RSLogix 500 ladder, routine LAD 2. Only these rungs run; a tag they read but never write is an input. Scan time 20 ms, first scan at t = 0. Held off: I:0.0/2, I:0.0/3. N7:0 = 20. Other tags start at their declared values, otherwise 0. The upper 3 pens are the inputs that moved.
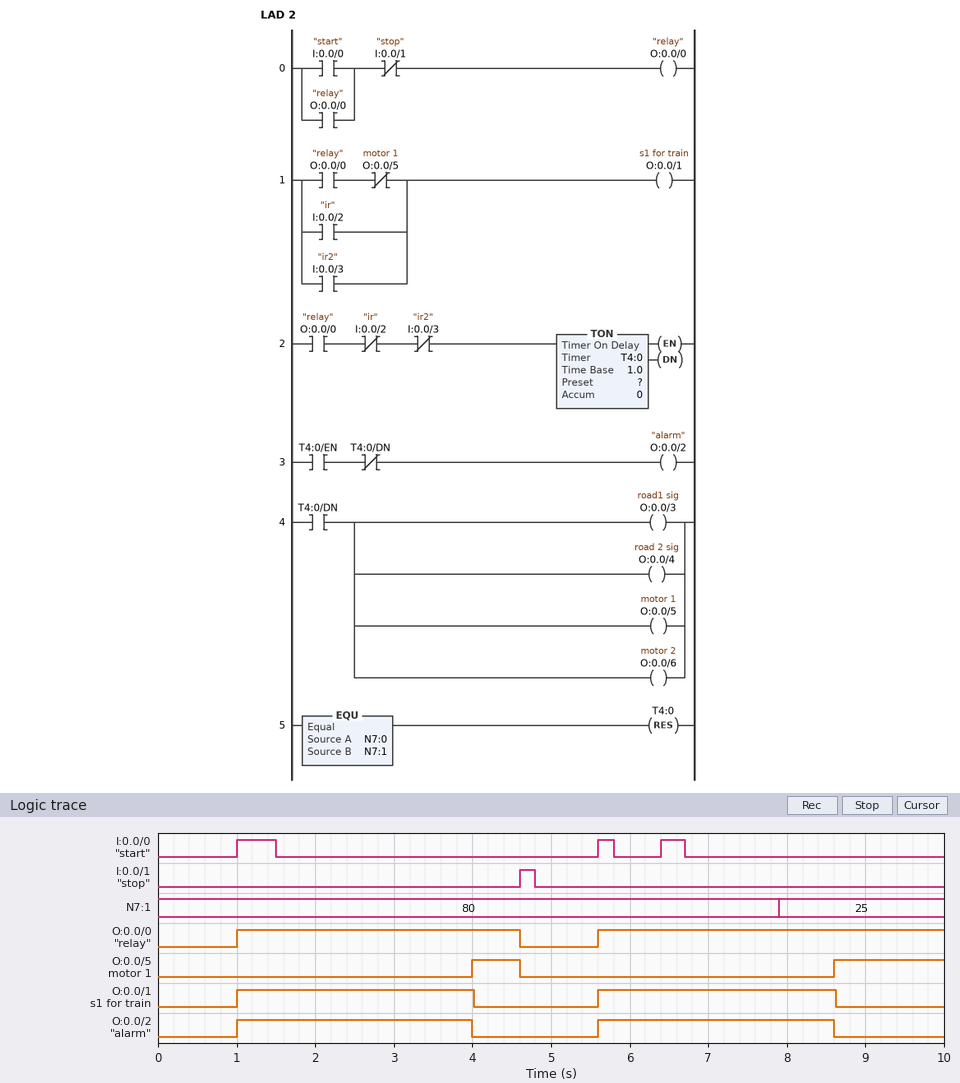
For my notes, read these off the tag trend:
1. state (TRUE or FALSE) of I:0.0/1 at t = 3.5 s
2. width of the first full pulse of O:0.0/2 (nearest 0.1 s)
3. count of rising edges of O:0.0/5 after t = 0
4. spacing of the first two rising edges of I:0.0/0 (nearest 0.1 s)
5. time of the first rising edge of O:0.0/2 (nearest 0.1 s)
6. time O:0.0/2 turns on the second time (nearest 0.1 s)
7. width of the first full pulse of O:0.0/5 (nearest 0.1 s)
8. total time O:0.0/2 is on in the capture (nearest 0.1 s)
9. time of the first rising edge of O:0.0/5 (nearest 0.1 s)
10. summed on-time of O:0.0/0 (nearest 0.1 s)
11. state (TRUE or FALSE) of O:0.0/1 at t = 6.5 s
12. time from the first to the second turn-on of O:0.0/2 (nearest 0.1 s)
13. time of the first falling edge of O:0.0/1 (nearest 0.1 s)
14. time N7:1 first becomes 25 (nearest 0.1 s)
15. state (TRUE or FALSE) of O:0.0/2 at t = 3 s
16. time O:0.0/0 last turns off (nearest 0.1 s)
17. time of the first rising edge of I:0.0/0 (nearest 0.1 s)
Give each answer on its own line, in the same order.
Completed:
FALSE
3.0 s
2
4.6 s
1.0 s
5.6 s
0.6 s
6.0 s
4.0 s
8.0 s
TRUE
4.6 s
4.0 s
7.9 s
TRUE
4.6 s
1.0 s
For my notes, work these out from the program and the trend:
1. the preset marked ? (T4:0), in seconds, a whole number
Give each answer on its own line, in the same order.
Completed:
3 s
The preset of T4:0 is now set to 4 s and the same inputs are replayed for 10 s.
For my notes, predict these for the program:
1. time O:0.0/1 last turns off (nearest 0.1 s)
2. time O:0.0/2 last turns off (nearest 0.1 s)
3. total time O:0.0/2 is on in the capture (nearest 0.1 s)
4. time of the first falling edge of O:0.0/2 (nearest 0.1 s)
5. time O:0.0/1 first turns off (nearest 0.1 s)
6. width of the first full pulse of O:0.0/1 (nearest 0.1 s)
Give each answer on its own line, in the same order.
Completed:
9.6 s
9.6 s
7.6 s
4.6 s
4.6 s
3.6 s
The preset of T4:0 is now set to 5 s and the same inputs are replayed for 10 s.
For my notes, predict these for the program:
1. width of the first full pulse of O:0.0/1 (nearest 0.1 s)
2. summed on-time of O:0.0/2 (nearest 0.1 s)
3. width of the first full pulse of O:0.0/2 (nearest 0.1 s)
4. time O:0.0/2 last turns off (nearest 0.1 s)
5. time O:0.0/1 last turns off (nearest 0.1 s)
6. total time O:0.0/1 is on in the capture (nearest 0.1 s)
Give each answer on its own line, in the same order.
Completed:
3.6 s
8.0 s
3.6 s
4.6 s
4.6 s
8.0 s
